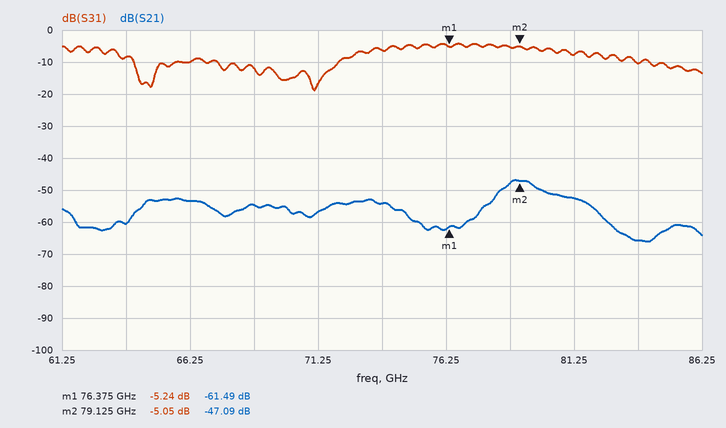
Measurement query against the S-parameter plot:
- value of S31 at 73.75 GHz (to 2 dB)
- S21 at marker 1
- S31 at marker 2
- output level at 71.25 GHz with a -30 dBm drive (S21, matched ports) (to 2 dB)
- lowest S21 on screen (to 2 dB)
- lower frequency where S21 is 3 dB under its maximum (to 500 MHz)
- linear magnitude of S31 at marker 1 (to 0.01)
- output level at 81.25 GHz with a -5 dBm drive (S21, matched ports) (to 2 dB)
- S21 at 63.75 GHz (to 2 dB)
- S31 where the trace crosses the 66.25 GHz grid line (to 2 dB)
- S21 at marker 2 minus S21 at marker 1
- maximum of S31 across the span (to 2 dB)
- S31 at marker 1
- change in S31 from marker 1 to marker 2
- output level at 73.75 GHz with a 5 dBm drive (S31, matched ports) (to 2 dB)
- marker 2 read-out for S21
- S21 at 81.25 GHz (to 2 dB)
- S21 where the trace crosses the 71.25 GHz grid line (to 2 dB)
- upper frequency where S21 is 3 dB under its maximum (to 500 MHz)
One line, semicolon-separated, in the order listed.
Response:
-6 dB; -61.49 dB; -5.05 dB; -86 dBm; -66 dB; 78.5 GHz; 0.55; -58 dBm; -60 dB; -10 dB; 14.40 dB; -4 dB; -5.24 dB; 0.19 dB; -2 dBm; -47.09 dB; -52 dB; -56 dB; 80.0 GHz
